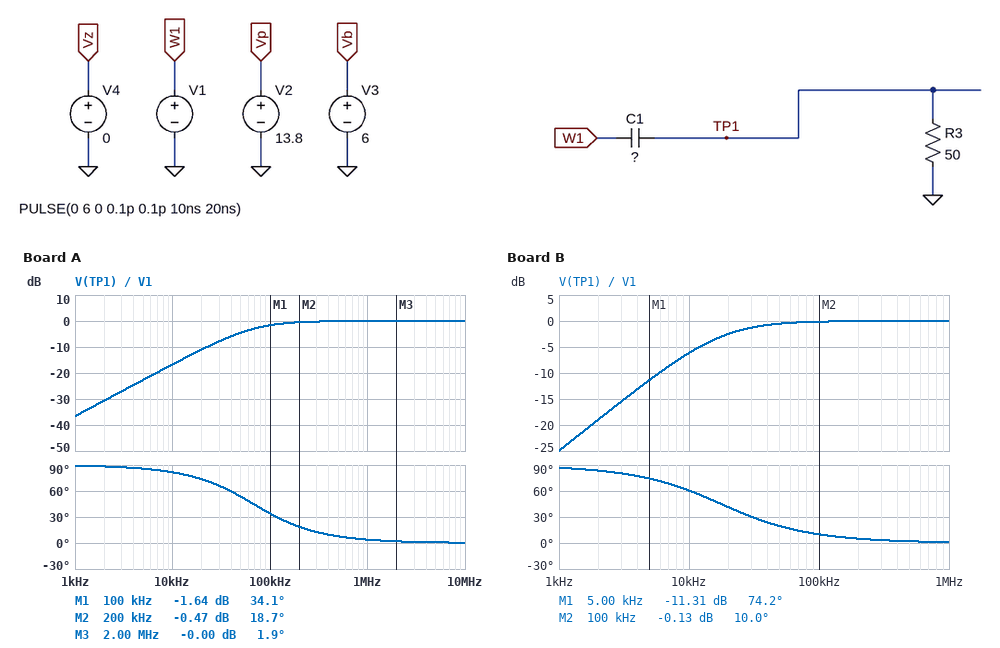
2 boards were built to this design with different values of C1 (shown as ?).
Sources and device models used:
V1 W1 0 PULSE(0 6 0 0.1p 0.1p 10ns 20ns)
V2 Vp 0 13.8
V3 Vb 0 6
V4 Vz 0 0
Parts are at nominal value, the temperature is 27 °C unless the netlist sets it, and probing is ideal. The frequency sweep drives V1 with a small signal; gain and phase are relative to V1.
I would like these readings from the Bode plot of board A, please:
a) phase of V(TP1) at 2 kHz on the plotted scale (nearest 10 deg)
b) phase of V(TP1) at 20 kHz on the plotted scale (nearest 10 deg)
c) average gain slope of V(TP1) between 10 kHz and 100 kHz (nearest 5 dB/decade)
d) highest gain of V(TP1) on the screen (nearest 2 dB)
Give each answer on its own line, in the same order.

90 deg
70 deg
15 dB/decade
0 dB
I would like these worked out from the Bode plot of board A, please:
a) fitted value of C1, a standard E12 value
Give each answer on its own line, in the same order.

47 nF
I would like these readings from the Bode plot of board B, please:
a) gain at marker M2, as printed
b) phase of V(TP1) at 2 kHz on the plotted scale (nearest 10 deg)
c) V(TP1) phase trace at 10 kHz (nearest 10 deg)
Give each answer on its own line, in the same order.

-0.13 dB
80 deg
60 deg
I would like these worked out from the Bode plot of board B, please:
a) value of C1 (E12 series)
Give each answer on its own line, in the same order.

180 nF
